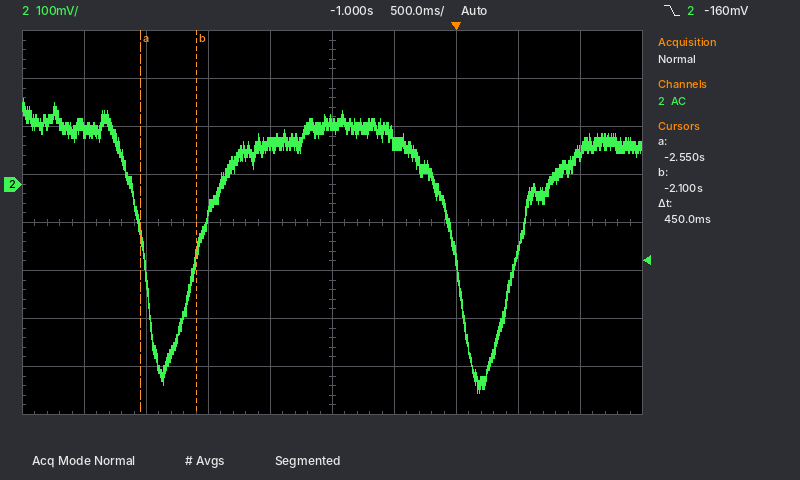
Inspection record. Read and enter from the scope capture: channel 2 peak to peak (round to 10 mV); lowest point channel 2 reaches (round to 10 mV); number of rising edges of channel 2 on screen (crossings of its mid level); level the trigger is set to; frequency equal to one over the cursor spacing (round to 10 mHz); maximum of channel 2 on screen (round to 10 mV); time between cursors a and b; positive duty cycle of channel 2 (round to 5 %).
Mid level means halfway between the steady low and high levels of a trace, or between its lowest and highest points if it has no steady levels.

610 mV
-430 mV
2
-160 mV
2.22 Hz
180 mV
450 ms
80 %
